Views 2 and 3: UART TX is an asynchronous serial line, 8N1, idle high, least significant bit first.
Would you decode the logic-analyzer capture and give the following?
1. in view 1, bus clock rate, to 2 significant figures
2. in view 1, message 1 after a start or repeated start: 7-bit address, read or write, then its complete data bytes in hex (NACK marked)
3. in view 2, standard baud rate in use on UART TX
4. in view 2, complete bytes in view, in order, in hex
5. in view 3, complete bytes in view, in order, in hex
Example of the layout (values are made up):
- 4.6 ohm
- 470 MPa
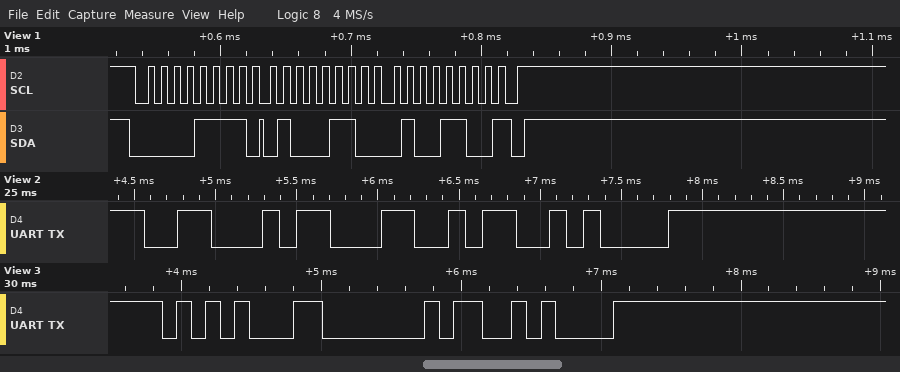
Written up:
- 100 kHz
- 0x07 read: 46 4C NACK
- 9600 baud
- 0x46 0x4C 0x0A
- 15 40 0A
